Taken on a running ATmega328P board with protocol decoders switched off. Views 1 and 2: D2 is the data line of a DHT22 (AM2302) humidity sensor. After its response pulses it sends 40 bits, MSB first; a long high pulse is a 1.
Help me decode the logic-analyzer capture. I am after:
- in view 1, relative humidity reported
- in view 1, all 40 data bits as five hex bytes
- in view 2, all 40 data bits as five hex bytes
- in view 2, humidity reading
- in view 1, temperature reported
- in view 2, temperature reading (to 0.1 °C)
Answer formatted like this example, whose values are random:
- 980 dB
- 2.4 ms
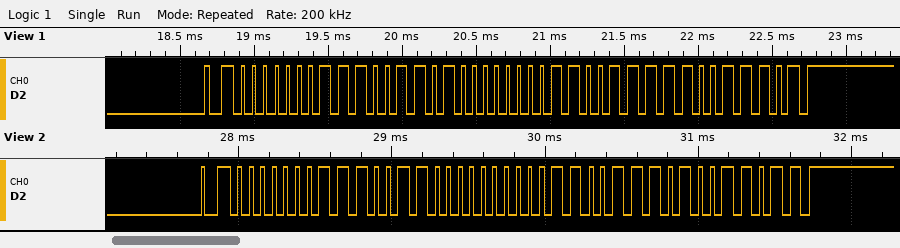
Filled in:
- 46.1 %
- 01 CD 00 CF 9D
- 01 CC 00 CE 9B
- 46.0 %
- 20.7 °C
- 20.6 °C
